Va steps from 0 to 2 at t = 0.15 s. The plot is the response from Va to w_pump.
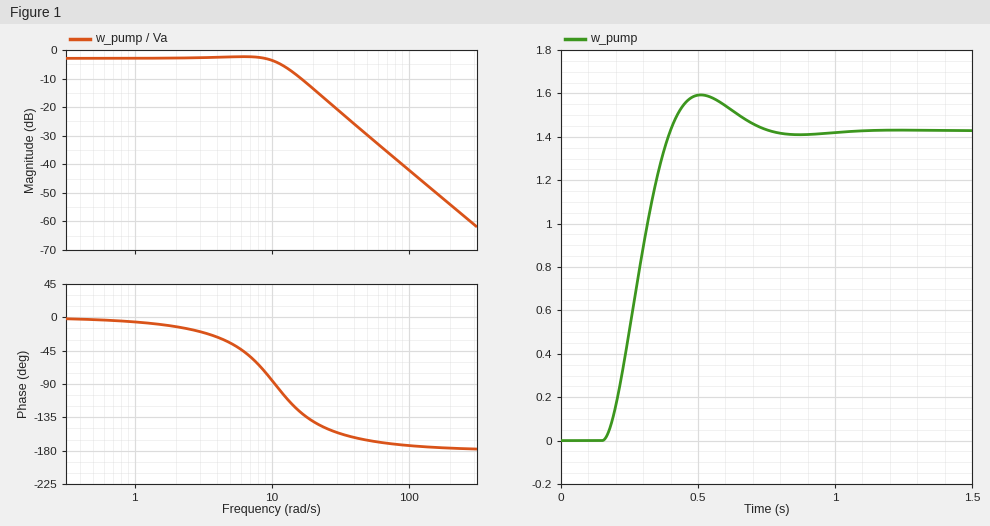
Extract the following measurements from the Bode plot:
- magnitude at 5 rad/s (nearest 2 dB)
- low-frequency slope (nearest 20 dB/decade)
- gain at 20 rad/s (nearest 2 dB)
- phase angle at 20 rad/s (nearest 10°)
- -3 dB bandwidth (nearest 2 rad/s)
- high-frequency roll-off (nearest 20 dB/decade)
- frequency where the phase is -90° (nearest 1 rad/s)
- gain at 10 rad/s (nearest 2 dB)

-2 dB
0 dB/decade
-14 dB
-140°
12 rad/s
-40 dB/decade
11 rad/s
-4 dB
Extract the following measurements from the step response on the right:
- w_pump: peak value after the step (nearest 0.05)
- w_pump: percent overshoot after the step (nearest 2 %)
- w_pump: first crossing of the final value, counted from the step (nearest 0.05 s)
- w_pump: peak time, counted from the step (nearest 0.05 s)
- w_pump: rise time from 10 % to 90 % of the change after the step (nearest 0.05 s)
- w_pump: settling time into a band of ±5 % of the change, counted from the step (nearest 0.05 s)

1.60
12 %
0.25 s
0.35 s
0.15 s
0.50 s
